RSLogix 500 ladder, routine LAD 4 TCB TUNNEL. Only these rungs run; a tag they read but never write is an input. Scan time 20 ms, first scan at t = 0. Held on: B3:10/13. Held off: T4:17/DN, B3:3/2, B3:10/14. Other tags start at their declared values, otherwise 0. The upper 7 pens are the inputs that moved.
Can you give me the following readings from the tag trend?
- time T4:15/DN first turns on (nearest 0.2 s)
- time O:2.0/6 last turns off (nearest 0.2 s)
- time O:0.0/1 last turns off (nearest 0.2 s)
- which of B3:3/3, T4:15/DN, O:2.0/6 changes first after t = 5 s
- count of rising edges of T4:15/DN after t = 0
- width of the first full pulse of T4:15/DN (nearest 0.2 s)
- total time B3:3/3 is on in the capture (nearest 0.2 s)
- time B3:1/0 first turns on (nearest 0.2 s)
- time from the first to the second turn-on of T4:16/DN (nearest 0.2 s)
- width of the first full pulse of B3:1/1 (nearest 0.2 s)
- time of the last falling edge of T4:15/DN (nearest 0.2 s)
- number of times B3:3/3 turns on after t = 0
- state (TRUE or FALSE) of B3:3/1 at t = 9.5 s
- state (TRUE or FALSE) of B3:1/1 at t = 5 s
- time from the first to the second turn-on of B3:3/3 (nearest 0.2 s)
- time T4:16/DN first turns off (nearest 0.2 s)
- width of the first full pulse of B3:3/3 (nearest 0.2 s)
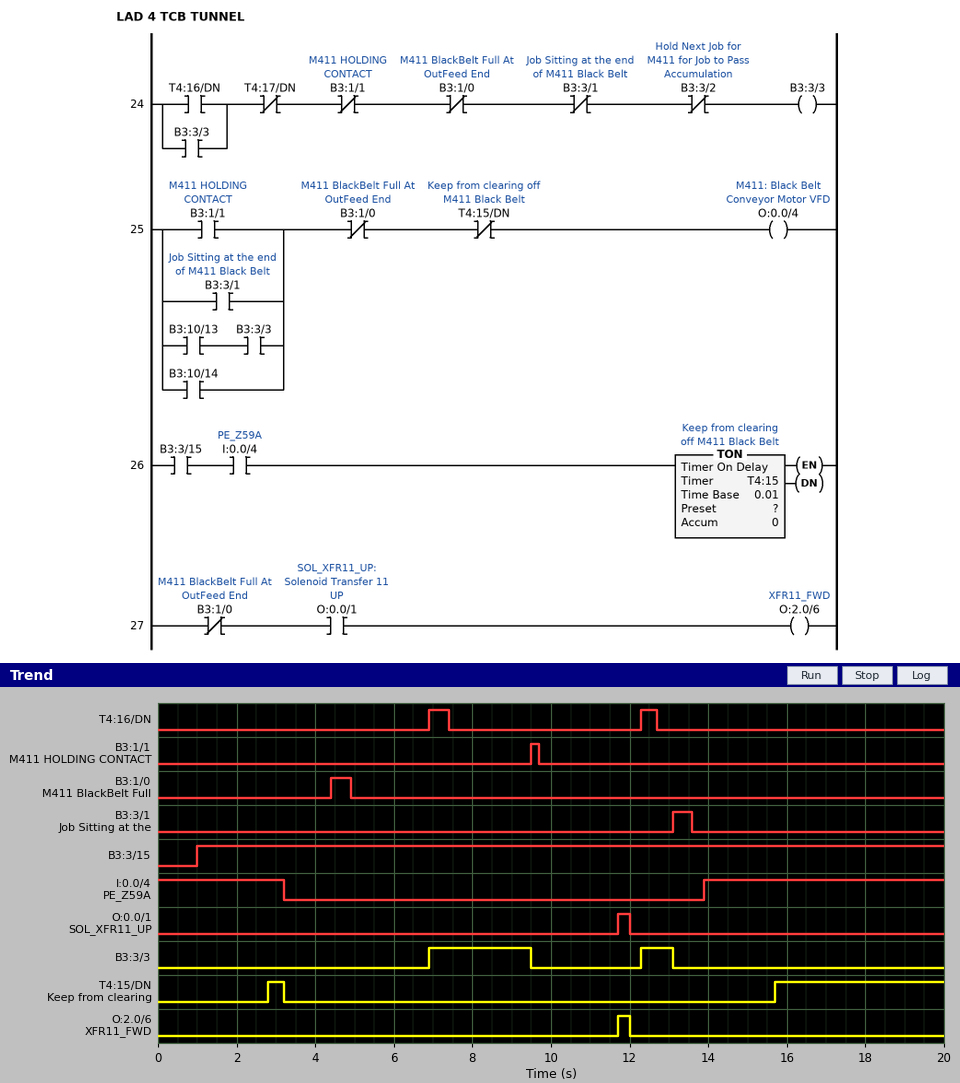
2.8 s
12.0 s
12.0 s
B3:3/3
2
0.4 s
3.4 s
4.4 s
5.4 s
0.2 s
3.2 s
2
FALSE
FALSE
5.4 s
7.4 s
2.6 s
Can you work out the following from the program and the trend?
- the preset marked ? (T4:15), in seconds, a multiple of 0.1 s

1.8 s
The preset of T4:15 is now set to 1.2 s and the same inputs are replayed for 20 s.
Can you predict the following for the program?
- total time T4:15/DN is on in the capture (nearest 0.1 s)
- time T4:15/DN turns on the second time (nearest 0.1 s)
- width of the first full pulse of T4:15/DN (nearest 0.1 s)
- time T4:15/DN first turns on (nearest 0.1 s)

5.9 s
15.1 s
1.0 s
2.2 s
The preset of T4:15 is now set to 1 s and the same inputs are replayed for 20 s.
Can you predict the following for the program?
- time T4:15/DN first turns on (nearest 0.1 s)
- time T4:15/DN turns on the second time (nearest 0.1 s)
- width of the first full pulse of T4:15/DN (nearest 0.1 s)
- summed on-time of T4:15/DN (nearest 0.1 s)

2.0 s
14.9 s
1.2 s
6.3 s
